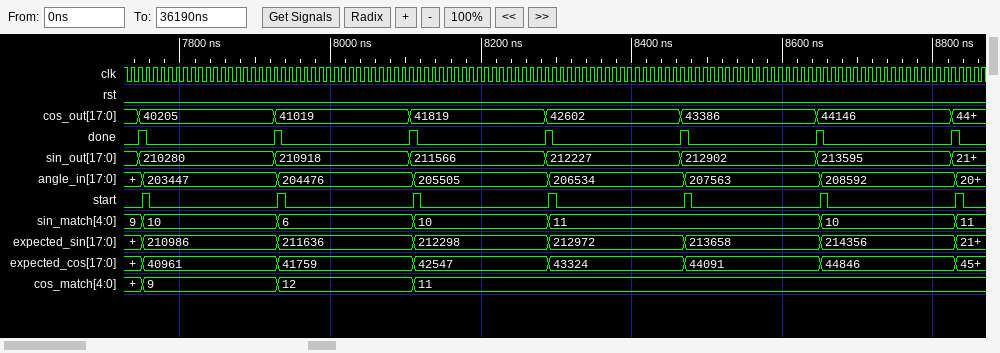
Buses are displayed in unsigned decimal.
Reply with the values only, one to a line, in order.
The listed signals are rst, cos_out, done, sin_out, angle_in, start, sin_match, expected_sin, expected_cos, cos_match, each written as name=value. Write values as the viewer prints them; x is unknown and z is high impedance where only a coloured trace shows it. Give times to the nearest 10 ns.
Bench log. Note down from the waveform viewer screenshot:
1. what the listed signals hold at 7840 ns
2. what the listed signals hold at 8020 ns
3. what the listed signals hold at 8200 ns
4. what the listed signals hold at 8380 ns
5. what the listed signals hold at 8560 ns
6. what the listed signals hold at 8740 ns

rst=0, cos_out=40205, done=0, sin_out=210280, angle_in=203447, start=0, sin_match=10, expected_sin=210986, expected_cos=40961, cos_match=9
rst=0, cos_out=41019, done=0, sin_out=210918, angle_in=204476, start=0, sin_match=6, expected_sin=211636, expected_cos=41759, cos_match=12
rst=0, cos_out=41819, done=0, sin_out=211566, angle_in=205505, start=0, sin_match=10, expected_sin=212298, expected_cos=42547, cos_match=11
rst=0, cos_out=42602, done=0, sin_out=212227, angle_in=206534, start=0, sin_match=11, expected_sin=212972, expected_cos=43324, cos_match=11
rst=0, cos_out=43386, done=0, sin_out=212902, angle_in=207563, start=0, sin_match=11, expected_sin=213658, expected_cos=44091, cos_match=11
rst=0, cos_out=44146, done=0, sin_out=213595, angle_in=208592, start=0, sin_match=10, expected_sin=214356, expected_cos=44846, cos_match=11
